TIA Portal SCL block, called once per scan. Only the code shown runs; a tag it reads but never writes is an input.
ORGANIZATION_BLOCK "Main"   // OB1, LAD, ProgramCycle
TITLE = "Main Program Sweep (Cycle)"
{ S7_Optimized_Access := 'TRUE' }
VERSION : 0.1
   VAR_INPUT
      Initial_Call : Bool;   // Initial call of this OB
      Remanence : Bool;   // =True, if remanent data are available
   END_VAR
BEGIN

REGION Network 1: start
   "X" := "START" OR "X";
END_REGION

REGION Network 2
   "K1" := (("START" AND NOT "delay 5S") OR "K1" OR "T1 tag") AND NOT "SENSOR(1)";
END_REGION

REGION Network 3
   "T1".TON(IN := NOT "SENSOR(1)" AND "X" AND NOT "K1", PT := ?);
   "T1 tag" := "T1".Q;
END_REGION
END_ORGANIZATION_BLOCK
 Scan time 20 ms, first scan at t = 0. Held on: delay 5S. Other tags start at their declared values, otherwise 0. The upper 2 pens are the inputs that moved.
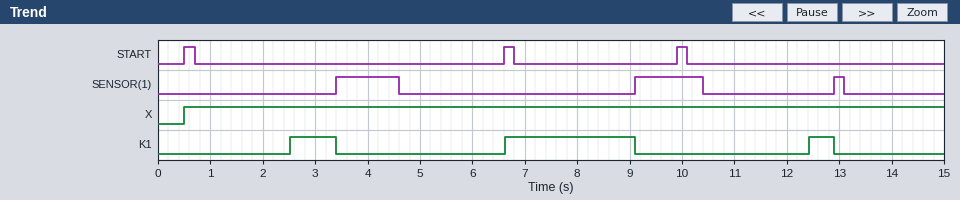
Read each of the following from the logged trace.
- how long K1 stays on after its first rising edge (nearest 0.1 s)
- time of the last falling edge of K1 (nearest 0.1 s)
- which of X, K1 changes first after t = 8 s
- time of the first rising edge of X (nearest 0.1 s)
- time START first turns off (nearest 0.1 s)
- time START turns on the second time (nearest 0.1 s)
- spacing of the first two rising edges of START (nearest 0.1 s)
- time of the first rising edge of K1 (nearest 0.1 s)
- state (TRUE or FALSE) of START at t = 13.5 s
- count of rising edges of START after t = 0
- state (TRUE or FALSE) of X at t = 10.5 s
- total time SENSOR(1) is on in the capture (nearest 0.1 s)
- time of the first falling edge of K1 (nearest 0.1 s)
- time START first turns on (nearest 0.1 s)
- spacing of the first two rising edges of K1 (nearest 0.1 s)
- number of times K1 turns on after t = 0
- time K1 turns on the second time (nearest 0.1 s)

0.9 s
12.9 s
K1
0.5 s
0.7 s
6.6 s
6.1 s
2.5 s
FALSE
3
TRUE
2.7 s
3.4 s
0.5 s
4.1 s
3
6.6 s
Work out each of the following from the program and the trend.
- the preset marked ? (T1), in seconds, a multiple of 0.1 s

2.0 s
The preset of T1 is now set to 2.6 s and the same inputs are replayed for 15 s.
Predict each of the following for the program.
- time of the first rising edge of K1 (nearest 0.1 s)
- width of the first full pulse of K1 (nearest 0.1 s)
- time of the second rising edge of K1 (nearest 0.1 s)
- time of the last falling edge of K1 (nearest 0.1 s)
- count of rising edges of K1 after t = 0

3.1 s
0.3 s
7.2 s
9.1 s
2
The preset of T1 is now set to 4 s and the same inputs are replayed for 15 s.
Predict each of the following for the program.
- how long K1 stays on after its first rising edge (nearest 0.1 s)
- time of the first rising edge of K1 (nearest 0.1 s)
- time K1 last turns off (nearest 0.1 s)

0.5 s
8.6 s
9.1 s
